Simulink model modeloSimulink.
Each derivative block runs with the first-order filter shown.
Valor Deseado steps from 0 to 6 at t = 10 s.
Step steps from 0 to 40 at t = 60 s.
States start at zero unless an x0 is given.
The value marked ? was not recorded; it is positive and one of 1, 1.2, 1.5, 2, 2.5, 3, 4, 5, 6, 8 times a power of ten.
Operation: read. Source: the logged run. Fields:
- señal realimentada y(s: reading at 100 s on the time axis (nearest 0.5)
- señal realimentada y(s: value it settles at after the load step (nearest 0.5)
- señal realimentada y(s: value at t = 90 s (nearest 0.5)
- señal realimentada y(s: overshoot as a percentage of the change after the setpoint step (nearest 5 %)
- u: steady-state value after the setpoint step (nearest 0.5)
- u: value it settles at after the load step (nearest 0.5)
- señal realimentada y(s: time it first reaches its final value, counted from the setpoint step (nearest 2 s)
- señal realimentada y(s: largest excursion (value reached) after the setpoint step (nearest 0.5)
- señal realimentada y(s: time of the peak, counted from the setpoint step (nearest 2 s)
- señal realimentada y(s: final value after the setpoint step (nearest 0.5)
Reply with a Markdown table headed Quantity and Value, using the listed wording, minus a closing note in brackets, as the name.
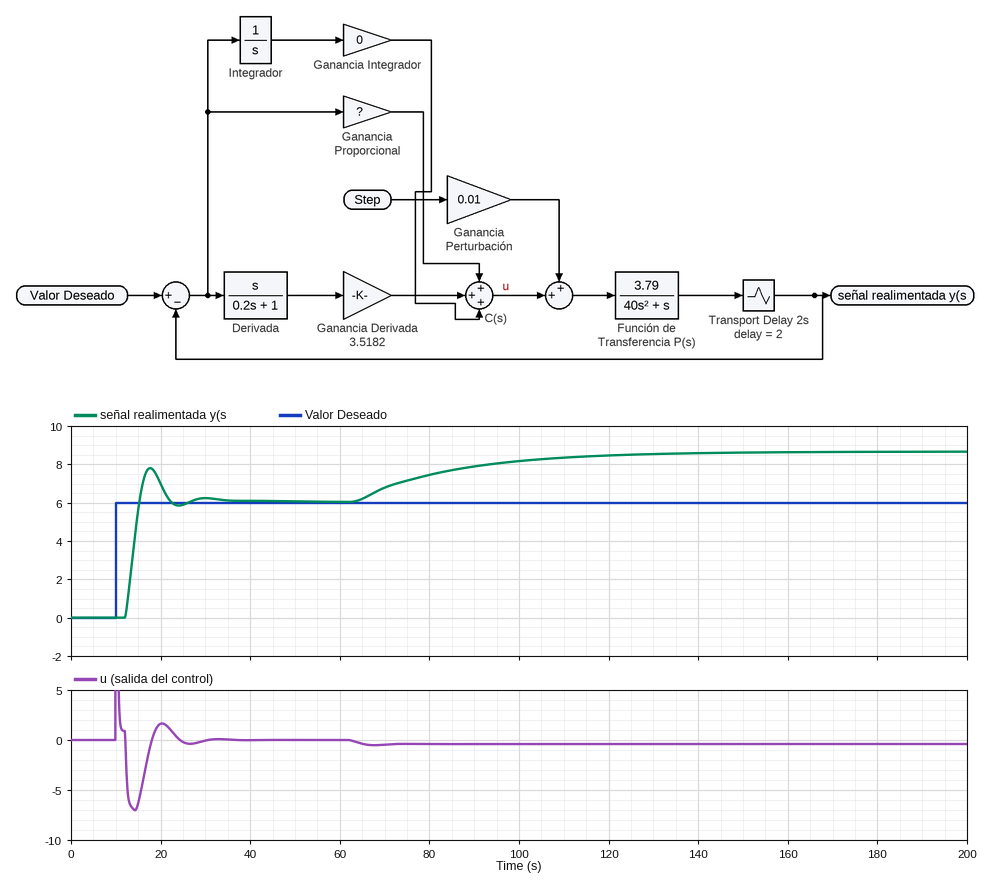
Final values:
| Quantity | Value |
|---|---|
| señal realimentada y(s: reading at 100 s on the time axis | 8.0 |
| señal realimentada y(s: value it settles at after the load step | 8.5 |
| señal realimentada y(s: value at t = 90 s | 8.0 |
| señal realimentada y(s: overshoot as a percentage of the change after the setpoint step | 30 % |
| u: steady-state value after the setpoint step | 0.0 |
| u: value it settles at after the load step | -0.5 |
| señal realimentada y(s: time it first reaches its final value, counted from the setpoint step | 6 s |
| señal realimentada y(s: largest excursion (value reached) after the setpoint step | 8.0 |
| señal realimentada y(s: time of the peak, counted from the setpoint step | 8 s |
| señal realimentada y(s: final value after the setpoint step | 6.0 |
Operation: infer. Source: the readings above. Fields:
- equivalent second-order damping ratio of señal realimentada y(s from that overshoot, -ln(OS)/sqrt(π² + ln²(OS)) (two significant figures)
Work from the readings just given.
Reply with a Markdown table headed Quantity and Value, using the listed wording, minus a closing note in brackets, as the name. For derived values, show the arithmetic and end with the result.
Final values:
| Quantity | Value |
|---|---|
| equivalent second-order damping ratio of señal realimentada y(s from that overshoot, -ln(OS)/sqrt(π² + ln²(OS)) | ln(0.3) = -1.204; 1.204 / sqrt(9.870 + 1.450) = 0.36 |
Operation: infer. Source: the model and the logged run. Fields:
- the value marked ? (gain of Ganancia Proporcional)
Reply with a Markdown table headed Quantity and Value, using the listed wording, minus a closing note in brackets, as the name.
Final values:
| Quantity | Value |
|---|---|
| the value marked ? | 0.15 |
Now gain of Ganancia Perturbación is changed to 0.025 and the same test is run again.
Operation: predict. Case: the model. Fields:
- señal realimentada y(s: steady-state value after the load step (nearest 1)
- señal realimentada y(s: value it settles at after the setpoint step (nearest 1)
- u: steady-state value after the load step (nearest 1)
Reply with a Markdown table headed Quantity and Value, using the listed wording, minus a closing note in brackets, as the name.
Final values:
| Quantity | Value |
|---|---|
| señal realimentada y(s: steady-state value after the load step | 13 |
| señal realimentada y(s: value it settles at after the setpoint step | 6 |
| u: steady-state value after the load step | -1 |
